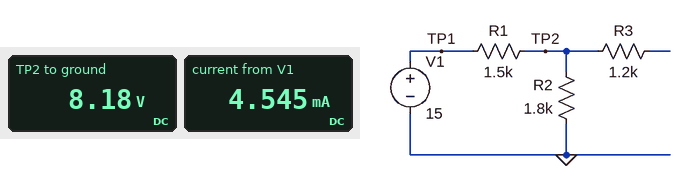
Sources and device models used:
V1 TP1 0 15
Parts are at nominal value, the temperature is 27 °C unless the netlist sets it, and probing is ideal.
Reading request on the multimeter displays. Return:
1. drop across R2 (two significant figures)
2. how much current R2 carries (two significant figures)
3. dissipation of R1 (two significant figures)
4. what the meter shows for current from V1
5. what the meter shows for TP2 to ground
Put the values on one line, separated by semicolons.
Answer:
8.2 V; 4.5 mA; 31 mW; 4.545 mA; 8.18 V
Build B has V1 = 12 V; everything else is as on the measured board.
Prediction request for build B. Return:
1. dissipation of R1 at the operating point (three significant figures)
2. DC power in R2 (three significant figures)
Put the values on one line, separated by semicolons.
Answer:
19.8 mW; 23.8 mW
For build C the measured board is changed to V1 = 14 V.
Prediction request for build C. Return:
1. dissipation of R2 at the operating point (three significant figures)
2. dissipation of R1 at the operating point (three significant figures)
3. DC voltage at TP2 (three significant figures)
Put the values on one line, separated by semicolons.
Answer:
32.4 mW; 27.0 mW; 7.64 V
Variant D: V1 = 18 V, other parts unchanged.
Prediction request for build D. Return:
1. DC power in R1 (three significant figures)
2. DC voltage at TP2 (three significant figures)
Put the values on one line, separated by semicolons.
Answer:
44.6 mW; 9.82 V
